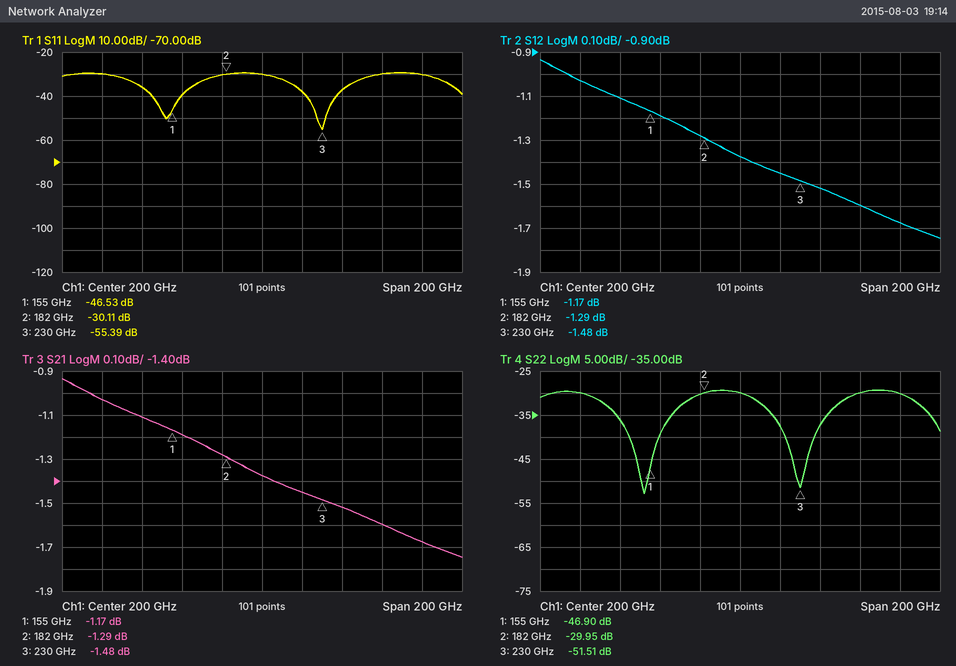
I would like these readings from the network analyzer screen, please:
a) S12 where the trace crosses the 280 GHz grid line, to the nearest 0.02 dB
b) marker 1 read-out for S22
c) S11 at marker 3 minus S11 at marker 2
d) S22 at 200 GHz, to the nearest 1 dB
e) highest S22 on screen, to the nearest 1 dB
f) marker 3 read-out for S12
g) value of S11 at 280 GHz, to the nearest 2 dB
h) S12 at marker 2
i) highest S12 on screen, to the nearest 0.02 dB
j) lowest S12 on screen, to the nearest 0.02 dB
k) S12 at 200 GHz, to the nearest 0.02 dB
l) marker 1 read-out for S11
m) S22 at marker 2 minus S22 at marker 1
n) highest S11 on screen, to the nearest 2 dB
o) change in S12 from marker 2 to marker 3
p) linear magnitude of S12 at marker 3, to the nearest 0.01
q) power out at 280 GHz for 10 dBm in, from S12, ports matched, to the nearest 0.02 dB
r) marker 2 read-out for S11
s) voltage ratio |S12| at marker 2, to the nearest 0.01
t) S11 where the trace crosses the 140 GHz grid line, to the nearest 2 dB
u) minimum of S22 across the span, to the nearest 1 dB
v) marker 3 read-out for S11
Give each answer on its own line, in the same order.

-1.68 dB
-46.90 dB
-25.28 dB
-30 dB
-29 dB
-1.48 dB
-30 dB
-1.29 dB
-0.94 dB
-1.74 dB
-1.38 dB
-46.53 dB
16.95 dB
-30 dB
-0.19 dB
0.84
8.32 dBm
-30.11 dB
0.86
-36 dB
-53 dB
-55.39 dB
